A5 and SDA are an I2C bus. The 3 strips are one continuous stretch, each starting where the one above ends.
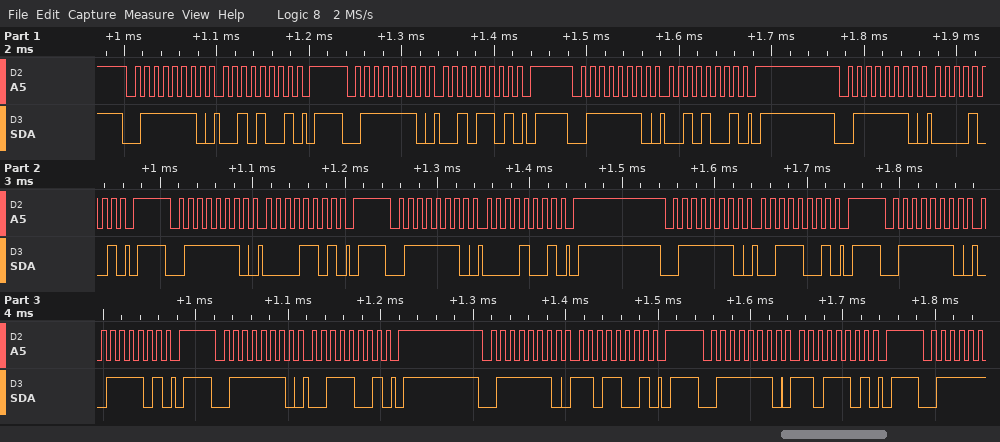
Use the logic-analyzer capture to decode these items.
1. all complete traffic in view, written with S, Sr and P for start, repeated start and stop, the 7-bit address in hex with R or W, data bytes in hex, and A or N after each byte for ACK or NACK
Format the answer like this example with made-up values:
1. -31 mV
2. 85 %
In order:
1. S 3FW A 29 A P S 3FW A 2D A P S 3FW A 29 A P S 3FW A 09 A P S 3FW A 0D A P S 3FW A 09 A P S 3FW A 39 A P S 3FW A 3D A P S 3FW A 39 A P S 3FW A D9 A P S 3FW A DD A P
